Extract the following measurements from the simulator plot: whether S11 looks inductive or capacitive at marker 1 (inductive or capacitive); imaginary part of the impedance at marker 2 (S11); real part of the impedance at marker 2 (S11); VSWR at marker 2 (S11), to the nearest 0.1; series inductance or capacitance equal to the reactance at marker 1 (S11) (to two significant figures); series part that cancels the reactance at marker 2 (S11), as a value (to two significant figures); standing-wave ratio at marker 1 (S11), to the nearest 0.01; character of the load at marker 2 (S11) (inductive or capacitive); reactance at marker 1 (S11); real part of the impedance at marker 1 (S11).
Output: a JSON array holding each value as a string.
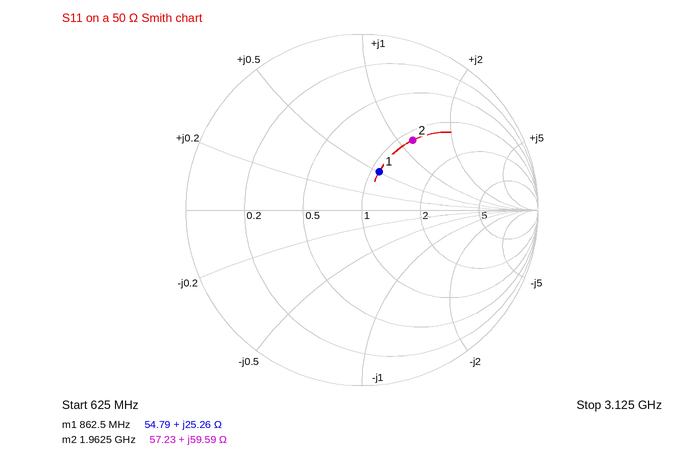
["inductive", "+59.59 Ω", "57.23 Ω", "2.9", "4.7 nH", "1.4 pF", "1.63", "inductive", "+25.26 Ω", "54.79 Ω"]
